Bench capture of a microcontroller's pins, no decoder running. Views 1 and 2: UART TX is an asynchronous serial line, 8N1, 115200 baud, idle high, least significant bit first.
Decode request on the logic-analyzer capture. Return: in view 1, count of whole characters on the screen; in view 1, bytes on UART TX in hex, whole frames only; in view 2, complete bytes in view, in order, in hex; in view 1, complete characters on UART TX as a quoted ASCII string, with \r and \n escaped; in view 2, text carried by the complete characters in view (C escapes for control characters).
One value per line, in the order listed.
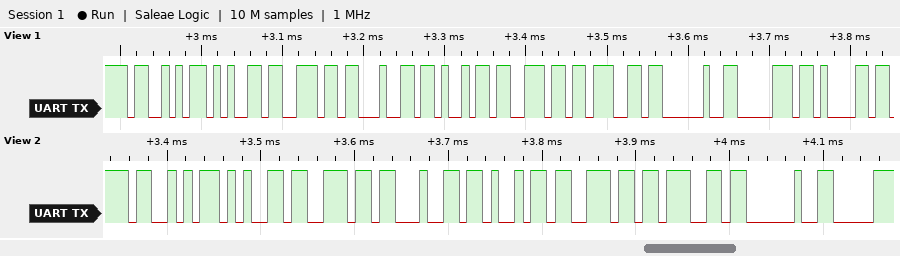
10
53 65 6E 64 69 6E 67 20 70 61
53 65 6E 64 69 6E 67 20
"Sending pa"
"Sending "
